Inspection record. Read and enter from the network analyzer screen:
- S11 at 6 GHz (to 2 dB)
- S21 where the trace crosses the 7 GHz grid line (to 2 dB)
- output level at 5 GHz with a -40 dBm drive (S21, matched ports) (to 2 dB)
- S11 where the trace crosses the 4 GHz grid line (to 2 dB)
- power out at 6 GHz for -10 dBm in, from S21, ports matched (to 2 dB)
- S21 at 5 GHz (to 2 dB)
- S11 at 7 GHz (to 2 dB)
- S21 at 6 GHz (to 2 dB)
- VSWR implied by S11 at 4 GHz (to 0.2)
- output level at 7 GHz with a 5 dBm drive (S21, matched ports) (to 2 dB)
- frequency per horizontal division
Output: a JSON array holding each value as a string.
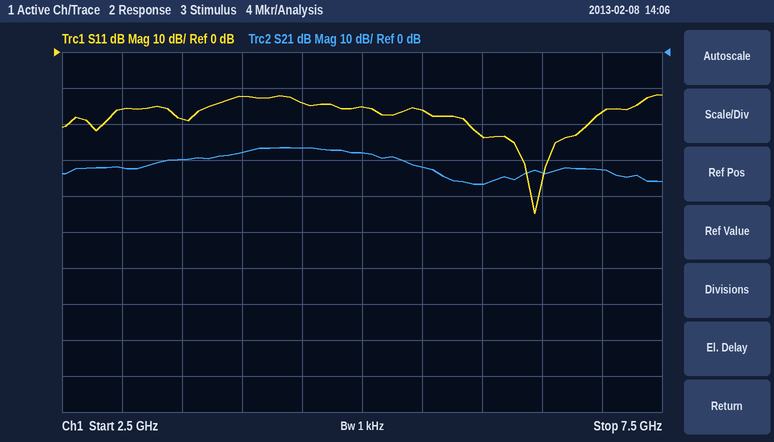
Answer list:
["-24 dB", "-32 dB", "-68 dBm", "-12 dB", "-46 dBm", "-28 dB", "-16 dB", "-36 dB", "1.6", "-28 dBm", "500 MHz"]
